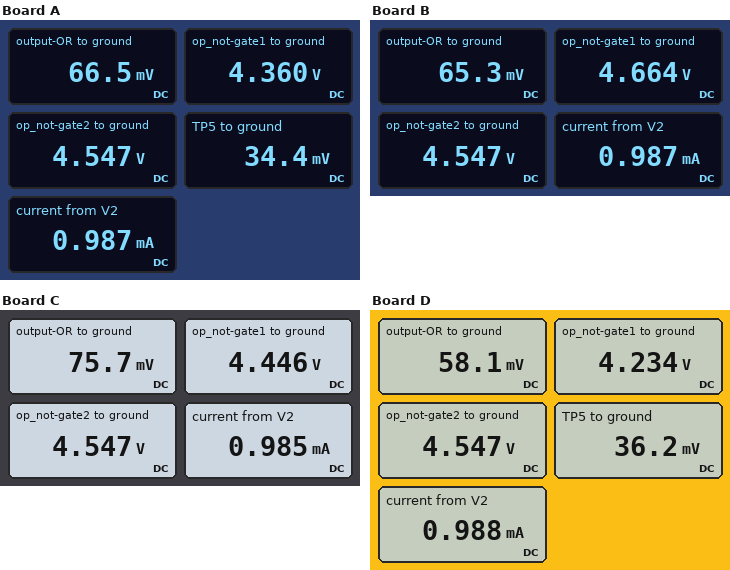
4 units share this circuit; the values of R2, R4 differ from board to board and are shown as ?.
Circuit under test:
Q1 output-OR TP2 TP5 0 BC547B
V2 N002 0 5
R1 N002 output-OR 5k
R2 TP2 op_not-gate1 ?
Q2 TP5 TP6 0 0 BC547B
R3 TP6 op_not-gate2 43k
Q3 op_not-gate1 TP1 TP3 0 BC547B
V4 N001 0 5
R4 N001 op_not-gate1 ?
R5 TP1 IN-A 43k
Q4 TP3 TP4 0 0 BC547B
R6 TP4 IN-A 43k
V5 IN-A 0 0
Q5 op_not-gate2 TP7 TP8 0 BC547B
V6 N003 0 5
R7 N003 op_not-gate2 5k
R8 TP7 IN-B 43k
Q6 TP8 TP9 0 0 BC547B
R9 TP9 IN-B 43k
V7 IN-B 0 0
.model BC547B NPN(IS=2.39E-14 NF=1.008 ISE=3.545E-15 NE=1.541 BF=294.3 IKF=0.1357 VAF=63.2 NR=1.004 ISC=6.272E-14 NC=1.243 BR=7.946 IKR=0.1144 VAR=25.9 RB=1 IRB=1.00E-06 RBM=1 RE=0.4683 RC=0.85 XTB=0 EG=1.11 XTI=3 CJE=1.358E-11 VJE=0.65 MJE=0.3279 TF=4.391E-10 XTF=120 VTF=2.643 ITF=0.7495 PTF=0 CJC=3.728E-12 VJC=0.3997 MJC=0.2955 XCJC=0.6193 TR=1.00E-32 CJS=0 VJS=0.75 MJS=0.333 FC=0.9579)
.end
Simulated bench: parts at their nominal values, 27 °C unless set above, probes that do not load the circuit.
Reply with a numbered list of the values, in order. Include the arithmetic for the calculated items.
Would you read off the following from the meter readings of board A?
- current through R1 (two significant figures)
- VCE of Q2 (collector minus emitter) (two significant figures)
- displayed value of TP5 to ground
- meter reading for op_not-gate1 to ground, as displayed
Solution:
1. (5 V - 66.5 mV) / 5 kΩ = 990 µA
2. 34.4 mV = 34 mV
3. 34.4 mV
4. 4.360 V
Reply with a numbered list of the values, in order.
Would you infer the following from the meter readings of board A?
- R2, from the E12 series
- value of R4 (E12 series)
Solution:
1. 39 kΩ
2. 6.8 kΩ
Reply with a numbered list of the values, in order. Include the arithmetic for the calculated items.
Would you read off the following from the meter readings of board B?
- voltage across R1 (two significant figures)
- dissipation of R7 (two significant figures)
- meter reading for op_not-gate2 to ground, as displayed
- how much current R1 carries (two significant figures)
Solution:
1. 5 V - 65.3 mV = 4.9 V
2. (5 V - 4.547 V)^2 / 5 kΩ = 41 µW
3. 4.547 V
4. (5 V - 65.3 mV) / 5 kΩ = 990 µA
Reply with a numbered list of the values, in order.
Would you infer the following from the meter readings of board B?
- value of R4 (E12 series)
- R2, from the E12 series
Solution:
1. 3.3 kΩ
2. 39 kΩ
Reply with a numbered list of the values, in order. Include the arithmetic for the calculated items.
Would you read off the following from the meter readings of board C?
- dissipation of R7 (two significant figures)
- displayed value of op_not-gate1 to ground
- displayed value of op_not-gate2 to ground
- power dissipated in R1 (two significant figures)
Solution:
1. (5 V - 4.547 V)^2 / 5 kΩ = 41 µW
2. 4.446 V
3. 4.547 V
4. (5 V - 75.7 mV)^2 / 5 kΩ = 4.8 mW
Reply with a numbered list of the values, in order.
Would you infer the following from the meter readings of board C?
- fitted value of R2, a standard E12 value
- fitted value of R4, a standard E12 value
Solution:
1. 68 kΩ
2. 10 kΩ
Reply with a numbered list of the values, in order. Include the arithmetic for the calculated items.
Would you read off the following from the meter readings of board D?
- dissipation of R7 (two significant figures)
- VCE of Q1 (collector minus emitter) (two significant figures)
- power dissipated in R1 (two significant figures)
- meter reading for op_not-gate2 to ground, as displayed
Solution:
1. (5 V - 4.547 V)^2 / 5 kΩ = 41 µW
2. 58.1 mV - 36.2 mV = 22 mV
3. (5 V - 58.1 mV)^2 / 5 kΩ = 4.9 mW
4. 4.547 V
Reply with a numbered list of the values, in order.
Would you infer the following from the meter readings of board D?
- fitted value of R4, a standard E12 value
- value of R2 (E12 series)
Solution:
1. 3.9 kΩ
2. 18 kΩ
